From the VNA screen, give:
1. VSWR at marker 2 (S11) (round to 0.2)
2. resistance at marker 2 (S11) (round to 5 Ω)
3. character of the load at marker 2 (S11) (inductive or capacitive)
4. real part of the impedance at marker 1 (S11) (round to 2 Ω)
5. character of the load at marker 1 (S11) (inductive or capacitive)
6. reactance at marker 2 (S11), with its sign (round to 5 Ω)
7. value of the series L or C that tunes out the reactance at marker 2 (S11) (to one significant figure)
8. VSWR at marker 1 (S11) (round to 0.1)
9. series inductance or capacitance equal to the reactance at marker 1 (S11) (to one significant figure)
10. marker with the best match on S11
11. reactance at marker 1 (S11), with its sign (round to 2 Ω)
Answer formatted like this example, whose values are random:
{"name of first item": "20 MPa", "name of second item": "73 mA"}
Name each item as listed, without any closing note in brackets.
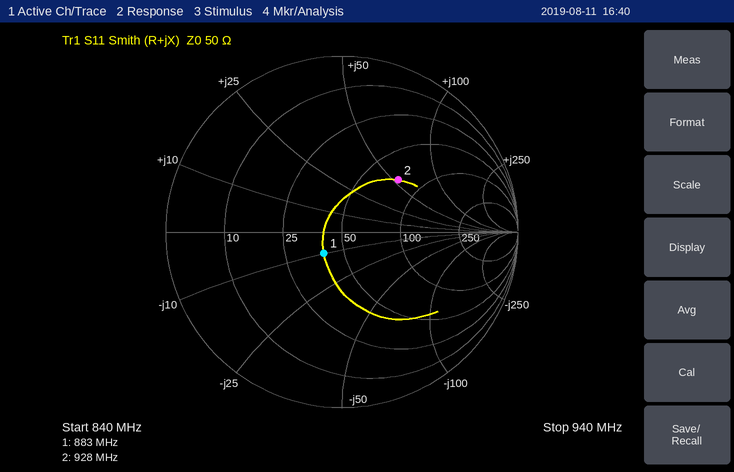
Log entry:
{"VSWR at marker 2 (S11)": "2.6", "resistance at marker 2 (S11)": "75 Ω", "character of the load at marker 2 (S11)": "inductive", "real part of the impedance at marker 1 (S11)": "40 Ω", "character of the load at marker 1 (S11)": "capacitive", "reactance at marker 2 (S11), with its sign": "+55 Ω", "value of the series L or C that tunes out the reactance at marker 2 (S11)": "3 pF", "VSWR at marker 1 (S11)": "1.4", "series inductance or capacitance equal to the reactance at marker 1 (S11)": "20 pF", "marker with the best match on S11": "marker 1", "reactance at marker 1 (S11), with its sign": "-10 Ω"}
